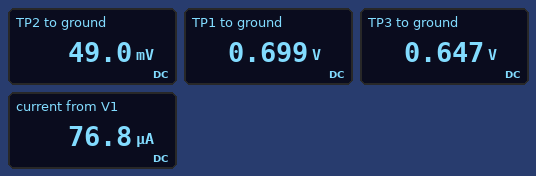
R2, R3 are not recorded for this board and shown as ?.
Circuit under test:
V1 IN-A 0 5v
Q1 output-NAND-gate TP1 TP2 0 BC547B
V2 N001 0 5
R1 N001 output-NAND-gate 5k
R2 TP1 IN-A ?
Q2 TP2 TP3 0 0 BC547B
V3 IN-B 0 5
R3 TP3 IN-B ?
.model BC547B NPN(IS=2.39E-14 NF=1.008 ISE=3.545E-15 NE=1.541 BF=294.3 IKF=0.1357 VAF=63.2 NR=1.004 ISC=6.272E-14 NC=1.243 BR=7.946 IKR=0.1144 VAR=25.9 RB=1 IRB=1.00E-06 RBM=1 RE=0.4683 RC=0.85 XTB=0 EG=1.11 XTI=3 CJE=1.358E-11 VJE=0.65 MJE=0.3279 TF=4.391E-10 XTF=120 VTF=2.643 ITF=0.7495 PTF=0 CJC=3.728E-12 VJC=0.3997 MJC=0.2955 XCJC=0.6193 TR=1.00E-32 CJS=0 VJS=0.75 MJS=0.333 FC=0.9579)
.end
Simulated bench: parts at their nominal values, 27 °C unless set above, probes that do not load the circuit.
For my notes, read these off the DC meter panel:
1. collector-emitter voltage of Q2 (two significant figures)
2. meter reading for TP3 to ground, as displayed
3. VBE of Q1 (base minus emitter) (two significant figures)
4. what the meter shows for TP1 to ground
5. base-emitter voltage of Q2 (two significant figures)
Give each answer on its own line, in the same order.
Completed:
49 mV
0.647 V
650 mV
0.699 V
650 mV
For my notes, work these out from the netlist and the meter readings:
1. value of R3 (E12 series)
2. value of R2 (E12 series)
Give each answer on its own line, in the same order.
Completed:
100 kΩ
56 kΩ
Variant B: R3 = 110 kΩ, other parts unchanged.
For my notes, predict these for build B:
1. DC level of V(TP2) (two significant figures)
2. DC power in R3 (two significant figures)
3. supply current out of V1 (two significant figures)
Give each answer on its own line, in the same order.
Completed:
51 mV
170 µW
77 µA
